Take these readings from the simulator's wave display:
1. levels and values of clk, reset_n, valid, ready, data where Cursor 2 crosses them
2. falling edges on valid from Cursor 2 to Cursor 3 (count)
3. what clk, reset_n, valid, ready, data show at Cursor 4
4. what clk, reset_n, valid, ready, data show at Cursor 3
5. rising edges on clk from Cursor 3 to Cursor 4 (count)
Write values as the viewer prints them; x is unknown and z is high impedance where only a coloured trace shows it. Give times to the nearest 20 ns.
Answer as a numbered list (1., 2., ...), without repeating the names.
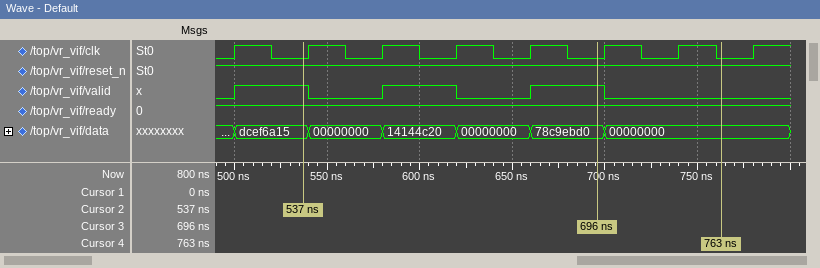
1. clk=0, reset_n=1, valid=1, ready=1, data=dcef6a15
2. 2
3. clk=0, reset_n=1, valid=0, ready=1, data=00000000
4. clk=0, reset_n=1, valid=1, ready=1, data=78c9ebd0
5. 2
